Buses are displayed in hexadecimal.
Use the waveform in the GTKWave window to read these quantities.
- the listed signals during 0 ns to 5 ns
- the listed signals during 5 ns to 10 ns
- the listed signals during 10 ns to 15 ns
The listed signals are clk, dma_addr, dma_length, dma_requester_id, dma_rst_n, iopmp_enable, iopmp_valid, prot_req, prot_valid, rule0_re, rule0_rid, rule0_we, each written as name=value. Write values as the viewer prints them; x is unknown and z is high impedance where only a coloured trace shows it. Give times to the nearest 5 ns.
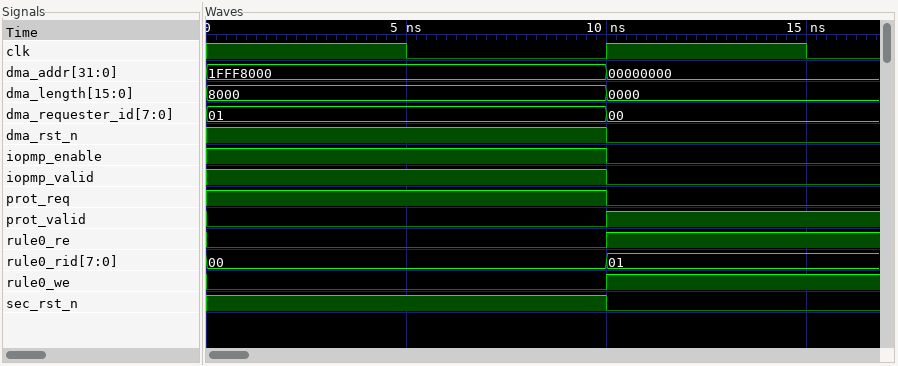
clk=1, dma_addr=1FFF8000, dma_length=8000, dma_requester_id=01, dma_rst_n=1, iopmp_enable=1, iopmp_valid=1, prot_req=1, prot_valid=0, rule0_re=0, rule0_rid=00, rule0_we=0
clk=0, dma_addr=1FFF8000, dma_length=8000, dma_requester_id=01, dma_rst_n=1, iopmp_enable=1, iopmp_valid=1, prot_req=1, prot_valid=0, rule0_re=0, rule0_rid=00, rule0_we=0
clk=1, dma_addr=00000000, dma_length=0000, dma_requester_id=00, dma_rst_n=0, iopmp_enable=0, iopmp_valid=0, prot_req=0, prot_valid=1, rule0_re=1, rule0_rid=01, rule0_we=1
